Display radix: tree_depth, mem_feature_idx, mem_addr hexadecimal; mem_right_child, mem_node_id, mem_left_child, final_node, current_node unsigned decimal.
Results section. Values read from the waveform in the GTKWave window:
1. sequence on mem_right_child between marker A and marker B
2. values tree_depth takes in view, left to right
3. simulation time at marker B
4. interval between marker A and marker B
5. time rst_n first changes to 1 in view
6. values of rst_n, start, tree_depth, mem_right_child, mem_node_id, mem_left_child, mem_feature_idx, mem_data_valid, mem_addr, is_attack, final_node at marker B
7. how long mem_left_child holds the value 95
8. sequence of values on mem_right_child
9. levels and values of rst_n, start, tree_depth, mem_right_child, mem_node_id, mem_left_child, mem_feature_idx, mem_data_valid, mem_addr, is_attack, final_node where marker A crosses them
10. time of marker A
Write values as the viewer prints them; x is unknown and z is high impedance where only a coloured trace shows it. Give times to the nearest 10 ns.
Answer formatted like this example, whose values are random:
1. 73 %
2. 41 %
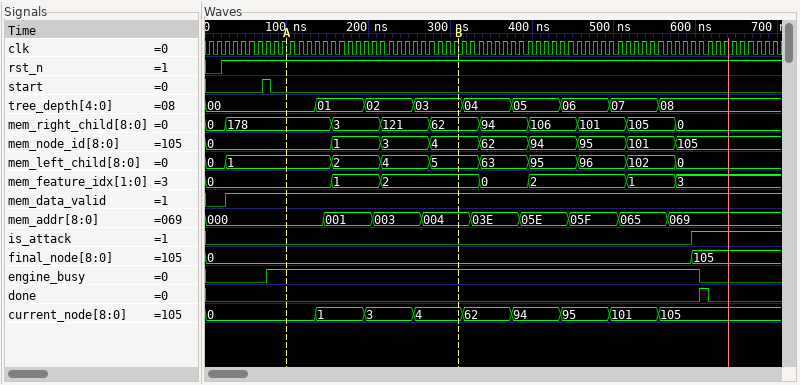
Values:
1. 178, 3, 121, 62
2. 00, 01, 02, 03, 04, 05, 06, 07, 08
3. 310 ns
4. 210 ns
5. 20 ns
6. rst_n=1, start=0, tree_depth=03, mem_right_child=62, mem_node_id=4, mem_left_child=5, mem_feature_idx=2, mem_data_valid=1, mem_addr=004, is_attack=0, final_node=0
7. 60 ns
8. 0, 178, 3, 121, 62, 94, 106, 101, 105, 0
9. rst_n=1, start=0, tree_depth=00, mem_right_child=178, mem_node_id=0, mem_left_child=1, mem_feature_idx=0, mem_data_valid=1, mem_addr=000, is_attack=0, final_node=0
10. 100 ns
